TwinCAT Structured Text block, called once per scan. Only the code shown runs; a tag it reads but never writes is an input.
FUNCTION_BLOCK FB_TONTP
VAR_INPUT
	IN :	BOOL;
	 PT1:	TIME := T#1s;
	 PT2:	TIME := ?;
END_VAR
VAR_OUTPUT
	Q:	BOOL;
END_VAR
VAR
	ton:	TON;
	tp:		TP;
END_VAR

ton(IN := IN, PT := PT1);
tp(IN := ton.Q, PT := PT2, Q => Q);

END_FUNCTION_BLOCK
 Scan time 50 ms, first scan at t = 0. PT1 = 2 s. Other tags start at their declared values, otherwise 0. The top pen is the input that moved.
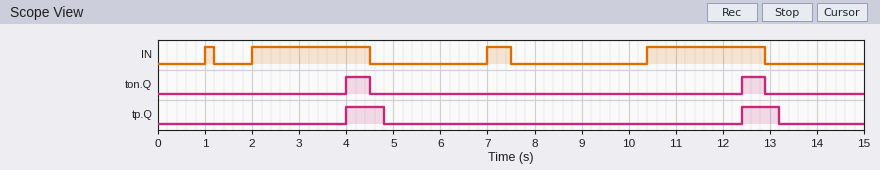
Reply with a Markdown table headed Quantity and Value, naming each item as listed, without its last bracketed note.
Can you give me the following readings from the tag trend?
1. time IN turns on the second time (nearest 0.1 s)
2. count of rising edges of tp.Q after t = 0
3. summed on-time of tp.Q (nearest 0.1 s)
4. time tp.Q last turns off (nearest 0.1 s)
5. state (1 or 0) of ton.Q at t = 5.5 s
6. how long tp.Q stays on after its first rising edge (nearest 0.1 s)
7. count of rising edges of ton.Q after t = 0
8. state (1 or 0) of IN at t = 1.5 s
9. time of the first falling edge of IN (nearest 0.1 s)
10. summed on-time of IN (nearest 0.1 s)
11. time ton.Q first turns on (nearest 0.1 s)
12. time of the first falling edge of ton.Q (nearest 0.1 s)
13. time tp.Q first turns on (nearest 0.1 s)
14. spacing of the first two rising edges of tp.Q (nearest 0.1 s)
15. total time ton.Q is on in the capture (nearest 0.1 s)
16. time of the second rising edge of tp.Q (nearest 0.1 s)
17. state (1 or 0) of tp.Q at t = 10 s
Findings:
| Quantity | Value |
|---|---|
| time IN turns on the second time | 2.0 s |
| count of rising edges of tp.Q after t = 0 | 2 |
| summed on-time of tp.Q | 1.6 s |
| time tp.Q last turns off | 13.2 s |
| state (1 or 0) of ton.Q at t = 5.5 s | 0 |
| how long tp.Q stays on after its first rising edge | 0.8 s |
| count of rising edges of ton.Q after t = 0 | 2 |
| state (1 or 0) of IN at t = 1.5 s | 0 |
| time of the first falling edge of IN | 1.2 s |
| summed on-time of IN | 5.7 s |
| time ton.Q first turns on | 4.0 s |
| time of the first falling edge of ton.Q | 4.5 s |
| time tp.Q first turns on | 4.0 s |
| spacing of the first two rising edges of tp.Q | 8.4 s |
| total time ton.Q is on in the capture | 1.0 s |
| time of the second rising edge of tp.Q | 12.4 s |
| state (1 or 0) of tp.Q at t = 10 s | 0 |
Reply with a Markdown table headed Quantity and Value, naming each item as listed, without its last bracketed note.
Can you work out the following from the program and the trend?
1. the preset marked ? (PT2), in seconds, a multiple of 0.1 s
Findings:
| Quantity | Value |
|---|---|
| the preset marked ? (PT2), in seconds, a multiple of 0.1 s | 0.8 s |
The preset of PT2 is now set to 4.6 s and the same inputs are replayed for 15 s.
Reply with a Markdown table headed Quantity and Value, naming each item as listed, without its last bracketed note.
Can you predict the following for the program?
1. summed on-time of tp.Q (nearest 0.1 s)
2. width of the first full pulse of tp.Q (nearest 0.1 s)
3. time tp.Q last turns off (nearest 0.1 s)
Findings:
| Quantity | Value |
|---|---|
| summed on-time of tp.Q | 7.2 s |
| width of the first full pulse of tp.Q | 4.6 s |
| time tp.Q last turns off | 8.6 s |
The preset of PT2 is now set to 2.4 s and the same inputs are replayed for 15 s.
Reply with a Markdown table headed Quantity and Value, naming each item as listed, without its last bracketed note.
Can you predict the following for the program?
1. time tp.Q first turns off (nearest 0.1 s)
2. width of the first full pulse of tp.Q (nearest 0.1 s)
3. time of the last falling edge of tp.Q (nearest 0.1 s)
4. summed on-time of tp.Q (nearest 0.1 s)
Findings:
| Quantity | Value |
|---|---|
| time tp.Q first turns off | 6.4 s |
| width of the first full pulse of tp.Q | 2.4 s |
| time of the last falling edge of tp.Q | 14.8 s |
| summed on-time of tp.Q | 4.8 s |
